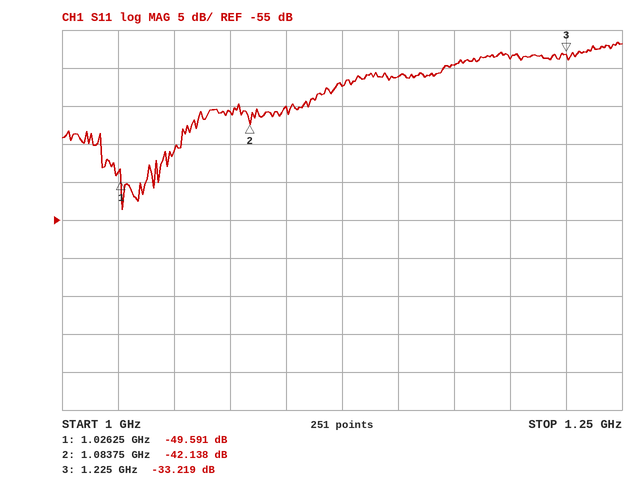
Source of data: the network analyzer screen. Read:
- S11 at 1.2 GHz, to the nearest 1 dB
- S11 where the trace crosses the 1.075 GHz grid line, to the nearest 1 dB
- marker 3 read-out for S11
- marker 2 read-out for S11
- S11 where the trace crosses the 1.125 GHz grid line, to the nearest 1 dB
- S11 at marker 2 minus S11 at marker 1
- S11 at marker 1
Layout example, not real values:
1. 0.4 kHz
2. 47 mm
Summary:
1. -34 dB
2. -41 dB
3. -33.219 dB
4. -42.138 dB
5. -37 dB
6. 7.453 dB
7. -49.591 dB
